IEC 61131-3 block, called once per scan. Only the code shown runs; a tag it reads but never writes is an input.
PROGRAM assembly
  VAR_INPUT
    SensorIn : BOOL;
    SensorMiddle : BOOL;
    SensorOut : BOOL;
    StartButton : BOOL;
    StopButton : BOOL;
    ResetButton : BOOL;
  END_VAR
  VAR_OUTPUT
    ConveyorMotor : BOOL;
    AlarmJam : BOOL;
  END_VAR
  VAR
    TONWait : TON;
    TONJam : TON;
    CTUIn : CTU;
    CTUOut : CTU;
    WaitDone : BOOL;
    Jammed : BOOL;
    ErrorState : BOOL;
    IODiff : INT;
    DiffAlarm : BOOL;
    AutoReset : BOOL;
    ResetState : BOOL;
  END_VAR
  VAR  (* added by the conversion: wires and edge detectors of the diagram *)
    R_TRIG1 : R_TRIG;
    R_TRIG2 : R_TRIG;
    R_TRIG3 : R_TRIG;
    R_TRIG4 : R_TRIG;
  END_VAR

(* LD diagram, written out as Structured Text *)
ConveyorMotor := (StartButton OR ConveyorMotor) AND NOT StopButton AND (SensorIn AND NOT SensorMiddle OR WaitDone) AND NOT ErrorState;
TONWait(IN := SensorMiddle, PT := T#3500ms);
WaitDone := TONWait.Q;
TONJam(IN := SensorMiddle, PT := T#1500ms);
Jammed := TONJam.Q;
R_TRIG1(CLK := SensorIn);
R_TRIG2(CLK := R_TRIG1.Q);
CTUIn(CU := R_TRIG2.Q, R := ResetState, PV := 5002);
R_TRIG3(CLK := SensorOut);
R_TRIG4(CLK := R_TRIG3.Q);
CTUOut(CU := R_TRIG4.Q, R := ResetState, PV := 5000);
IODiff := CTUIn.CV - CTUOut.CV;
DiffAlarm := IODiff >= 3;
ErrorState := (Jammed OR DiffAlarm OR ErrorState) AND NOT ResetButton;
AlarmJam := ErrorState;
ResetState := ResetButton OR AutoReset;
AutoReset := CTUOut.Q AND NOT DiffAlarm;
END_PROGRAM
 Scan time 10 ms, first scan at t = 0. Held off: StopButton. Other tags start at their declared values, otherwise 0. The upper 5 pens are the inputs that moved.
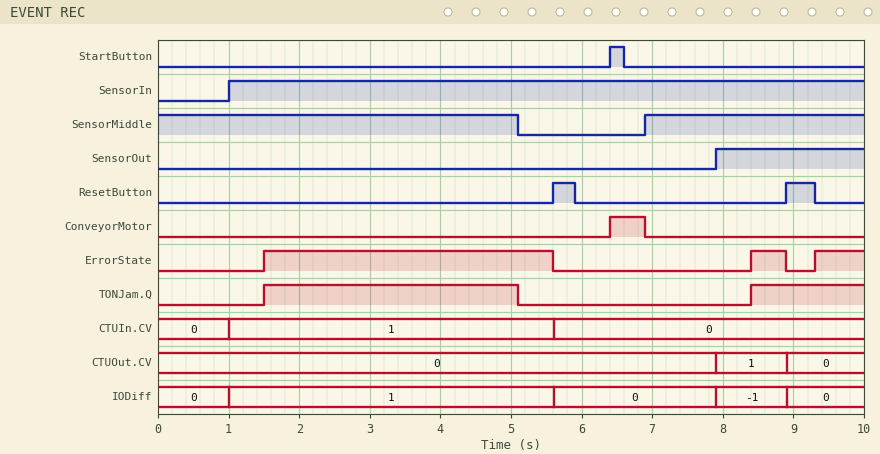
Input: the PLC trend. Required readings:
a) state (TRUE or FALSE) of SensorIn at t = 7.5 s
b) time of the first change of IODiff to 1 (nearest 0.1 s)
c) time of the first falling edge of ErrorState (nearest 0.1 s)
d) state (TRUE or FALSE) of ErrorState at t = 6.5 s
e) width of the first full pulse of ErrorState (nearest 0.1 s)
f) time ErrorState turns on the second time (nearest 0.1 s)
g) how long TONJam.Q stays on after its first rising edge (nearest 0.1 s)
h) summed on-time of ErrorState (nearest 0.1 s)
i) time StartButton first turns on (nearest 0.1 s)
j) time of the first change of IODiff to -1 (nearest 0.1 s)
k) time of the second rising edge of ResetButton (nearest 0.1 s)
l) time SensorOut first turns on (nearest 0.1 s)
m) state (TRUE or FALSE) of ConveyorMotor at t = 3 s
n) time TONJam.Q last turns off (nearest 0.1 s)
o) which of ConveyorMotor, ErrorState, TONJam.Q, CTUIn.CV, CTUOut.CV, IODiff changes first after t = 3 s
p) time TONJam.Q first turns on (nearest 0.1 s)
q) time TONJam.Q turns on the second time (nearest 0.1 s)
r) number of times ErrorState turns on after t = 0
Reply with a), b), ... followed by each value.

a) TRUE
b) 1.0 s
c) 5.6 s
d) FALSE
e) 4.1 s
f) 8.4 s
g) 3.6 s
h) 5.3 s
i) 6.4 s
j) 7.9 s
k) 8.9 s
l) 7.9 s
m) FALSE
n) 5.1 s
o) TONJam.Q
p) 1.5 s
q) 8.4 s
r) 3
